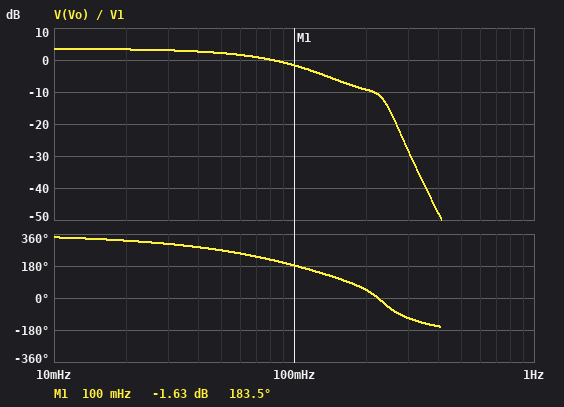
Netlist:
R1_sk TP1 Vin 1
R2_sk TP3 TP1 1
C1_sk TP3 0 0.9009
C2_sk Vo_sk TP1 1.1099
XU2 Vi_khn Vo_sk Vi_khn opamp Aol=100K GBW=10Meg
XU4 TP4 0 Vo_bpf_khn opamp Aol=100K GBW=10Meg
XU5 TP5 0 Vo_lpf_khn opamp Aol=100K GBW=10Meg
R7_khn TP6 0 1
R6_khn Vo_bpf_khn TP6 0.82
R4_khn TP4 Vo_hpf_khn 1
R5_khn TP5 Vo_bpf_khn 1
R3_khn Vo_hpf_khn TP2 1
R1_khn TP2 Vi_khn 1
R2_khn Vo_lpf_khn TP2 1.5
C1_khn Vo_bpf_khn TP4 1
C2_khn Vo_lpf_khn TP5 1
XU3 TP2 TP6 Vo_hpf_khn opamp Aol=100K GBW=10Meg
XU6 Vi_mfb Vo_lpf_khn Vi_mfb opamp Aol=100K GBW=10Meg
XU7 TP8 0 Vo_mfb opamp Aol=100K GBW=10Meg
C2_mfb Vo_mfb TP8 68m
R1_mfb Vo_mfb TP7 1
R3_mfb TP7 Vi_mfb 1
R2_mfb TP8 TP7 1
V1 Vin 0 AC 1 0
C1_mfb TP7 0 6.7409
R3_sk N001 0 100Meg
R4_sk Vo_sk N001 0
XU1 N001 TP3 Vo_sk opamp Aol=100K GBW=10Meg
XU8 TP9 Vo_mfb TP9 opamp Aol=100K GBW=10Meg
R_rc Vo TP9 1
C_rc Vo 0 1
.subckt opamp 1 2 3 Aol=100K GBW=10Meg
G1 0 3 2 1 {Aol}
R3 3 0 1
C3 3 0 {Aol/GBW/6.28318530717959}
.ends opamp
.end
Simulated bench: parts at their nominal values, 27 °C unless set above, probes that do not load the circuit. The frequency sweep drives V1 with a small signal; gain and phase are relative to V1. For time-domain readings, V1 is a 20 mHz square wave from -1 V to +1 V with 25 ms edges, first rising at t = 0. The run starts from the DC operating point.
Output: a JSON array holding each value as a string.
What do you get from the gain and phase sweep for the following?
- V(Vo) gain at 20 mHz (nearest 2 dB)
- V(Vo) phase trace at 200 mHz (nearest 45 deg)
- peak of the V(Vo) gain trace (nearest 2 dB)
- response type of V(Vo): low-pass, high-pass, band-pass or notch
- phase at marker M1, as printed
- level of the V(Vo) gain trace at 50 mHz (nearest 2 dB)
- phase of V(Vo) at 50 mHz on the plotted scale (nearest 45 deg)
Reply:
["4 dB", "45 deg", "4 dB", "low-pass", "183.5 deg", "2 dB", "270 deg"]
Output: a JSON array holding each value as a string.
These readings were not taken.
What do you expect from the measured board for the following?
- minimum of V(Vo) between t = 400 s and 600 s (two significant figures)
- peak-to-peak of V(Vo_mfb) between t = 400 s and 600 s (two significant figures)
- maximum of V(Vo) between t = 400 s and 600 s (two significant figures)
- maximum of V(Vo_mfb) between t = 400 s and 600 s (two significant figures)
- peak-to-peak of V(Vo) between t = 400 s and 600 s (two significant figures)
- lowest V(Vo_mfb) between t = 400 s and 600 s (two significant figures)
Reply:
["-1.5 V", "3.1 V", "1.5 V", "1.5 V", "3.0 V", "-1.5 V"]
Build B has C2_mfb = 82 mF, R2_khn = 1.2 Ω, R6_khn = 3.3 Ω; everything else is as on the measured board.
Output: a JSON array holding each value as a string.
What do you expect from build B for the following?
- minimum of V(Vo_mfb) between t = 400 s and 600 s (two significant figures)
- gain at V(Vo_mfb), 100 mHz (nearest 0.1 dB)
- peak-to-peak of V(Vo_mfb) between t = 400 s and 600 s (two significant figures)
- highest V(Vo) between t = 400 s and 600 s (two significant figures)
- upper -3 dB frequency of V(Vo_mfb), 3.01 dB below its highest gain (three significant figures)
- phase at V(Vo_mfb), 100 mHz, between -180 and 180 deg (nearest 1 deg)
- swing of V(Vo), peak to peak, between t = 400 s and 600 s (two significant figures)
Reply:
["-2.1 V", "4.2 dB", "4.1 V", "1.7 V", "192 mHz", "-116 deg", "3.5 V"]
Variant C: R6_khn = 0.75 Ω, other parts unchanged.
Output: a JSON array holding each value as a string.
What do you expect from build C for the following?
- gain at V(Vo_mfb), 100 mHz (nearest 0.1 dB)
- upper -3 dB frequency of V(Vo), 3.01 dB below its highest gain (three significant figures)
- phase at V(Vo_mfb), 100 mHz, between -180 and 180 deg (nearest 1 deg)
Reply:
["-0.5 dB", "71.8 mHz", "-145 deg"]
